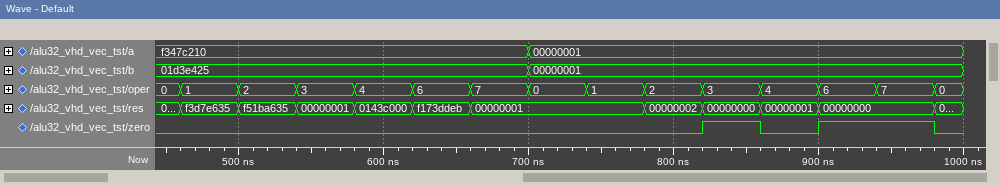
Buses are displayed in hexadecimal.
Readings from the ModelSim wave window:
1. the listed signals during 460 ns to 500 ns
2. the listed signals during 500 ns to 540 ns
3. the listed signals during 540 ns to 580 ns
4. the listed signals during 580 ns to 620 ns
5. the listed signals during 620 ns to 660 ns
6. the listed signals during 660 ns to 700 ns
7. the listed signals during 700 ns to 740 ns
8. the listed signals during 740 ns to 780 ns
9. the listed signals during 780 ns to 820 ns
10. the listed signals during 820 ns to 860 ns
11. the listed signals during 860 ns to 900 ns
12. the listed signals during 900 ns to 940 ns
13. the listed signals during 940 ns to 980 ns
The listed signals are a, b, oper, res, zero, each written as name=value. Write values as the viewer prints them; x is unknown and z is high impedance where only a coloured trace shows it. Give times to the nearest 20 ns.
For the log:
a=f347c210, b=01d3e425, oper=1, res=f3d7e635, zero=0
a=f347c210, b=01d3e425, oper=2, res=f51ba635, zero=0
a=f347c210, b=01d3e425, oper=3, res=00000001, zero=0
a=f347c210, b=01d3e425, oper=4, res=0143c000, zero=0
a=f347c210, b=01d3e425, oper=6, res=f173ddeb, zero=0
a=f347c210, b=01d3e425, oper=7, res=00000001, zero=0
a=00000001, b=00000001, oper=0, res=00000001, zero=0
a=00000001, b=00000001, oper=1, res=00000001, zero=0
a=00000001, b=00000001, oper=2, res=00000002, zero=0
a=00000001, b=00000001, oper=3, res=00000000, zero=1
a=00000001, b=00000001, oper=4, res=00000001, zero=0
a=00000001, b=00000001, oper=6, res=00000000, zero=1
a=00000001, b=00000001, oper=7, res=00000000, zero=1
